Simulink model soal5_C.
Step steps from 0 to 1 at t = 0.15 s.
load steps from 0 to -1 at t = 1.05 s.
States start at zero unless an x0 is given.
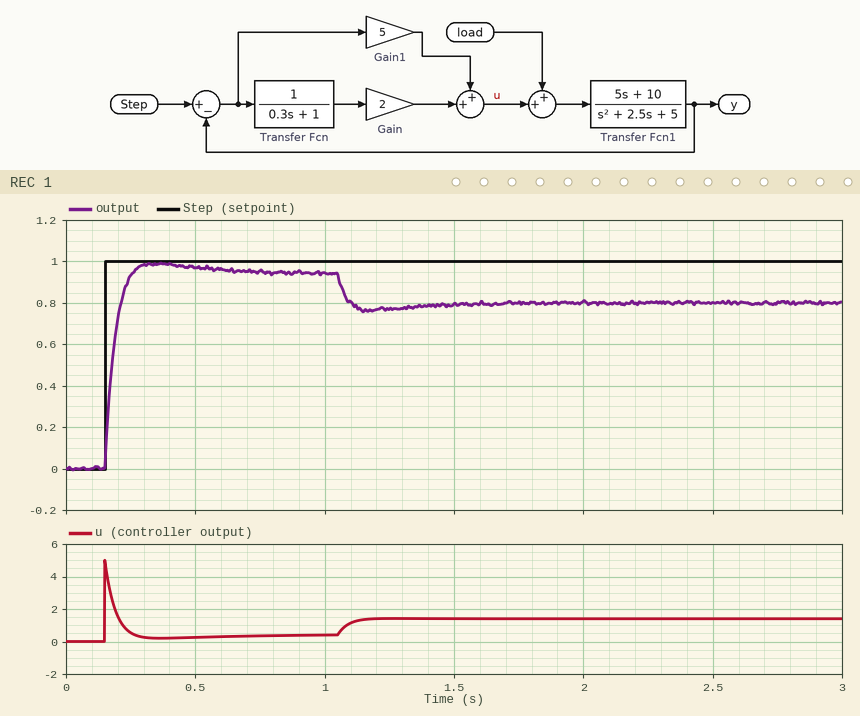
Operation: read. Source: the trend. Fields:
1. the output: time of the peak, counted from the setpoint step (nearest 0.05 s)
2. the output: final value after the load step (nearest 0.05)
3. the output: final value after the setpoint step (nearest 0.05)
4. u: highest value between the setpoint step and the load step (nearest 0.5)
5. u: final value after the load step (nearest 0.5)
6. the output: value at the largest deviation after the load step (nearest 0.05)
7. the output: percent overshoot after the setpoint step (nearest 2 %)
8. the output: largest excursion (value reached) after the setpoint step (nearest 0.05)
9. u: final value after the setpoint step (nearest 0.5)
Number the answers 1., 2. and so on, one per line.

1. 0.20 s
2. 0.80
3. 0.95
4. 5.0
5. 1.5
6. 0.75
7. 6 %
8. 1.00
9. 0.5
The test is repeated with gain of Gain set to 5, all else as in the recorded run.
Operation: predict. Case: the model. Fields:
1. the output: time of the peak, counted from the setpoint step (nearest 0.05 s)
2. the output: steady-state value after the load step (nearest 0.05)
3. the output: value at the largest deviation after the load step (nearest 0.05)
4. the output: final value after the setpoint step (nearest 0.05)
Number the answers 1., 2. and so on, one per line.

1. 0.15 s
2. 0.85
3. 0.80
4. 0.95
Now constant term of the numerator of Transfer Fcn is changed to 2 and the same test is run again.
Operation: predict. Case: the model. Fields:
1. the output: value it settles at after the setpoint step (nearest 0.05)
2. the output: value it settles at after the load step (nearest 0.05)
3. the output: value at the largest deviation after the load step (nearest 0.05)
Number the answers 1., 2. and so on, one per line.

1. 0.95
2. 0.85
3. 0.80
